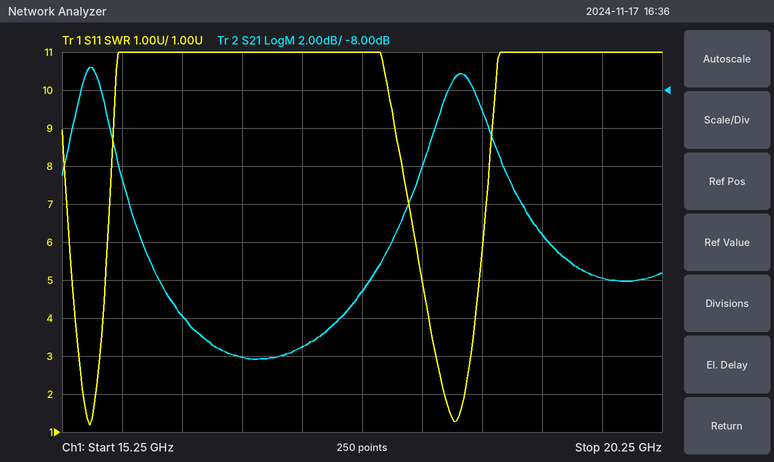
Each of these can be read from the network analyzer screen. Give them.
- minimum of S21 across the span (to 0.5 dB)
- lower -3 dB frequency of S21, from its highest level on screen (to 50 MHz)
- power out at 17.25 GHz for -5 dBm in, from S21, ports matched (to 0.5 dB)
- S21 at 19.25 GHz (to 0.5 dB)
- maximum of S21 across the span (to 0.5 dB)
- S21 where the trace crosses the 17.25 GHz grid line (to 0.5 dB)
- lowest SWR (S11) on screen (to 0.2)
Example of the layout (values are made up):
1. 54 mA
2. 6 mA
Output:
1. -22.0 dB
2. 15.35 GHz
3. -26.5 dBm
4. -15.5 dB
5. -7.0 dB
6. -21.5 dB
7. 1.2
